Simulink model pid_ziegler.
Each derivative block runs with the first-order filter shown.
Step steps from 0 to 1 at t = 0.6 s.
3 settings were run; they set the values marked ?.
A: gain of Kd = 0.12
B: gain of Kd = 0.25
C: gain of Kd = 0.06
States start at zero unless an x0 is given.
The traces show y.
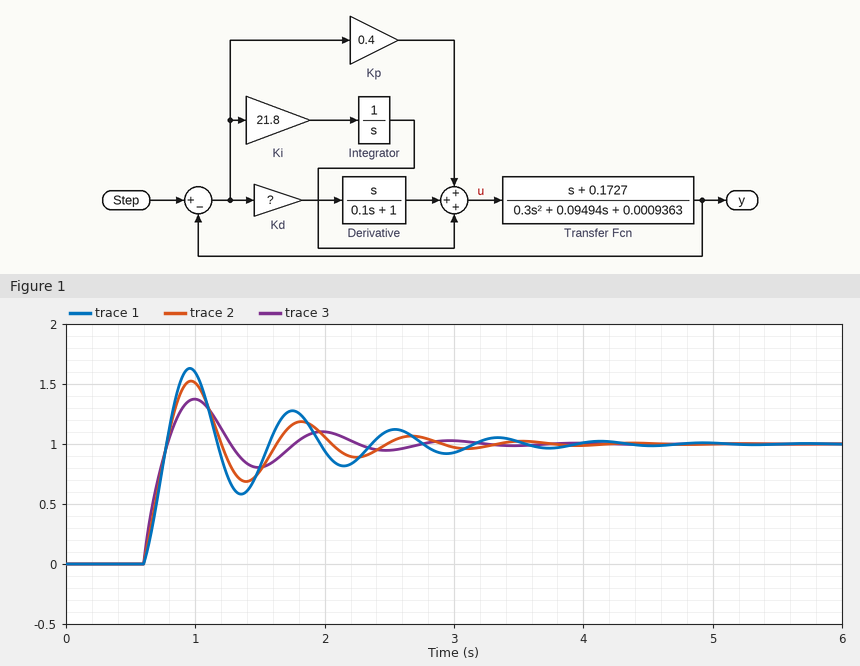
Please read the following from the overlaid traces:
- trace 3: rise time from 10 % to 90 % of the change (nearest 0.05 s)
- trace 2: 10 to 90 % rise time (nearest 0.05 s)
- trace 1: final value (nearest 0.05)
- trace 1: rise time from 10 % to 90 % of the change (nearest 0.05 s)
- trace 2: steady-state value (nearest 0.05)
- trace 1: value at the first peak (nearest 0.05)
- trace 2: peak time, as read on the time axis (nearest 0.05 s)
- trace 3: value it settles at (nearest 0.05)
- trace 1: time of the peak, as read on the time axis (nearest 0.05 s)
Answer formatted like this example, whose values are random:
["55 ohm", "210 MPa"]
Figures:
["0.15 s", "0.15 s", "1.00", "0.15 s", "1.00", "1.65", "0.95 s", "1.00", "0.95 s"]
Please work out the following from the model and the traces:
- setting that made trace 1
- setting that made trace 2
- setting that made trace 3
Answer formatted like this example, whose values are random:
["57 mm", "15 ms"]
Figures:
["C", "A", "B"]
